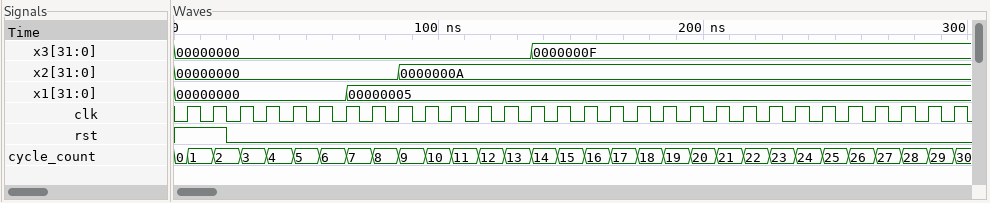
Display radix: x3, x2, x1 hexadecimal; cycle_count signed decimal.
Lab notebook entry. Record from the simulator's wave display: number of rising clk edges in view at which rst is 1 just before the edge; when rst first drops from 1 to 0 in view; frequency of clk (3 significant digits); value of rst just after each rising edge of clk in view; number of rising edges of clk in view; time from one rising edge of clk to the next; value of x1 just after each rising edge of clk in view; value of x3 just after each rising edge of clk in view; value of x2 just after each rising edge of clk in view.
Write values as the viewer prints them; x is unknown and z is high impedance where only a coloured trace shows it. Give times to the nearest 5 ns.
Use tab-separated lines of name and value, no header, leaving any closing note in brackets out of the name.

number of rising clk edges in view at which rst is 1 just before the edge	2
when rst first drops from 1 to 0 in view	20 ns
frequency of clk	100 MHz
value of rst just after each rising edge of clk in view	1 1 0 0 0 0 0 0 0 0 0 0 0 0 0 0 0 0 0 0 0 0 0 0 0 0 0 0 0 0
number of rising edges of clk in view	30
time from one rising edge of clk to the next	10 ns
value of x1 just after each rising edge of clk in view	00000000, 00000000, 00000000, 00000000, 00000000, 00000000, 00000005, 00000005, 00000005, 00000005, 00000005, 00000005, 00000005, 00000005, 00000005, 00000005, 00000005, 00000005, 00000005, 00000005, 00000005, 00000005, 00000005, 00000005, 00000005, 00000005, 00000005, 00000005, 00000005, 00000005
value of x3 just after each rising edge of clk in view	00000000, 00000000, 00000000, 00000000, 00000000, 00000000, 00000000, 00000000, 00000000, 00000000, 00000000, 00000000, 00000000, 0000000F, 0000000F, 0000000F, 0000000F, 0000000F, 0000000F, 0000000F, 0000000F, 0000000F, 0000000F, 0000000F, 0000000F, 0000000F, 0000000F, 0000000F, 0000000F, 0000000F
value of x2 just after each rising edge of clk in view	00000000, 00000000, 00000000, 00000000, 00000000, 00000000, 00000000, 00000000, 0000000A, 0000000A, 0000000A, 0000000A, 0000000A, 0000000A, 0000000A, 0000000A, 0000000A, 0000000A, 0000000A, 0000000A, 0000000A, 0000000A, 0000000A, 0000000A, 0000000A, 0000000A, 0000000A, 0000000A, 0000000A, 0000000A
